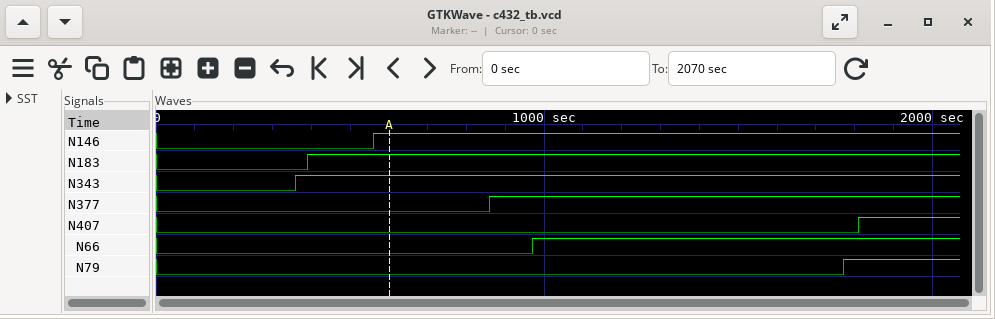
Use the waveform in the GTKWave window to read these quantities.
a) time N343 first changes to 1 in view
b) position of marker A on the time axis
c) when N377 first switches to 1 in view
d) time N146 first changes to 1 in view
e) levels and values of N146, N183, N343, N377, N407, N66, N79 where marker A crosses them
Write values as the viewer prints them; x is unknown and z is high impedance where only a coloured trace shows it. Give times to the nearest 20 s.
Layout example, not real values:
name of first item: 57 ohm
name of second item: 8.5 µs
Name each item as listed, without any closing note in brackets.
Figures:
time N343 first changes to 1 in view: 360 s
position of marker A on the time axis: 600 s
when N377 first switches to 1 in view: 860 s
time N146 first changes to 1 in view: 560 s
levels and values of N146, N183, N343, N377, N407, N66, N79 where marker A crosses them: N146=1, N183=1, N343=1, N377=0, N407=0, N66=0, N79=0
